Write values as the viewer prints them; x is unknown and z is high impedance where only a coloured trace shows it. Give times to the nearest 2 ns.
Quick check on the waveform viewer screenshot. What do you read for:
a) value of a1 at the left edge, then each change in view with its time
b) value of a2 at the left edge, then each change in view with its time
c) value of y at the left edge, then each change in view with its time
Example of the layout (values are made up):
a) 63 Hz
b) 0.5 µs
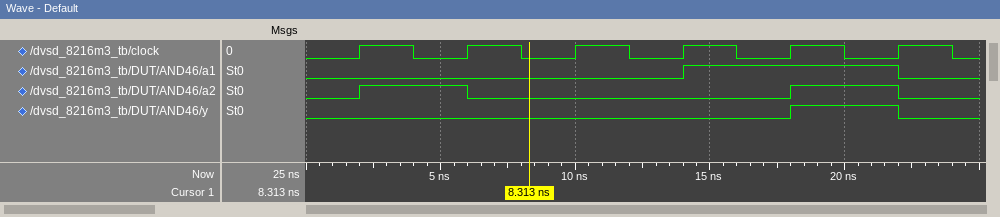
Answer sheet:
a) 0, 1 at 14 ns, 0 at 22 ns
b) 0, 1 at 2 ns, 0 at 6 ns, 1 at 18 ns, 0 at 22 ns
c) 0, 1 at 18 ns, 0 at 22 ns
